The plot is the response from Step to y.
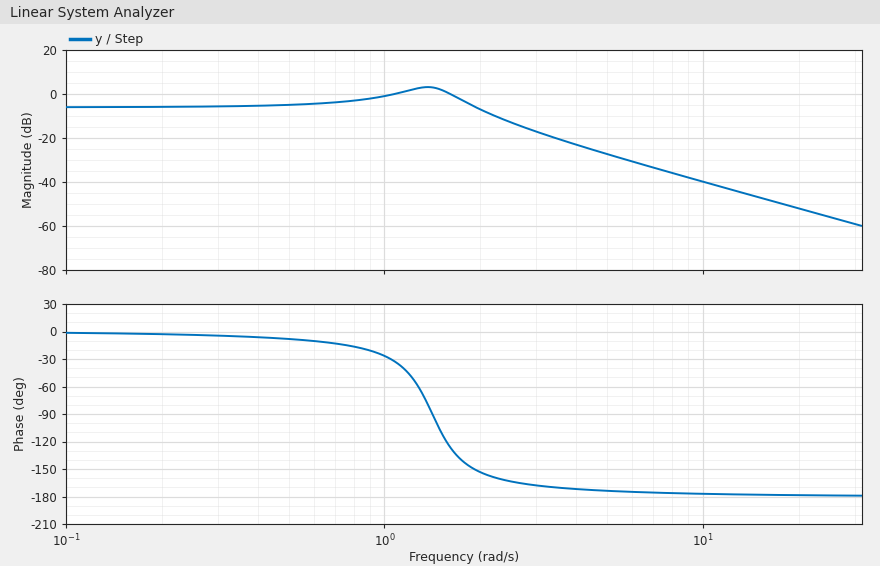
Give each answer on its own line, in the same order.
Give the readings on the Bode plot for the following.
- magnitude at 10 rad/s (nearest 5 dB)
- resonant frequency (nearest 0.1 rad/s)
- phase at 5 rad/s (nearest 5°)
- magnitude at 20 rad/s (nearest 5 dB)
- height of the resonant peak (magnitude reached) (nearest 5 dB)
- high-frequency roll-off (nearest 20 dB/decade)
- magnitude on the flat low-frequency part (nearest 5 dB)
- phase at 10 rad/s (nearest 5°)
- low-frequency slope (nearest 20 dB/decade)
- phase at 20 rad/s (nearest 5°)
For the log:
-40 dB
1.4 rad/s
-175°
-50 dB
5 dB
-40 dB/decade
-5 dB
-175°
0 dB/decade
-180°
